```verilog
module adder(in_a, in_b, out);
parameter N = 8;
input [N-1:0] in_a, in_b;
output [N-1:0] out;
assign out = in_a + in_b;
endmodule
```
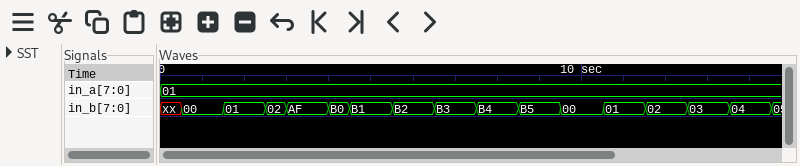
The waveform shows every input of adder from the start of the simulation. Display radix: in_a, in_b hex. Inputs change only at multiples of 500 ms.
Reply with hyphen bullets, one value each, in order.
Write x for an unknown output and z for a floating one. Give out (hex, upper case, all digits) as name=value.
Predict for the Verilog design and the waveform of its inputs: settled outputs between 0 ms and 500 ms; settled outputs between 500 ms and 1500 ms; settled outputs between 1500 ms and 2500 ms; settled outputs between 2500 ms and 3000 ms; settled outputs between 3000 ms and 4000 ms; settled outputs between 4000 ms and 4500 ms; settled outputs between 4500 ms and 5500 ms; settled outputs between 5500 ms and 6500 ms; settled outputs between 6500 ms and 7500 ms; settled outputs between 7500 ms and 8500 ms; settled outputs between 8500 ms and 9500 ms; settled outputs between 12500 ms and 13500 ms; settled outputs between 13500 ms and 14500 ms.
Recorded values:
- out=x
- out=01
- out=02
- out=03
- out=B0
- out=B1
- out=B2
- out=B3
- out=B4
- out=B5
- out=B6
- out=04
- out=05
